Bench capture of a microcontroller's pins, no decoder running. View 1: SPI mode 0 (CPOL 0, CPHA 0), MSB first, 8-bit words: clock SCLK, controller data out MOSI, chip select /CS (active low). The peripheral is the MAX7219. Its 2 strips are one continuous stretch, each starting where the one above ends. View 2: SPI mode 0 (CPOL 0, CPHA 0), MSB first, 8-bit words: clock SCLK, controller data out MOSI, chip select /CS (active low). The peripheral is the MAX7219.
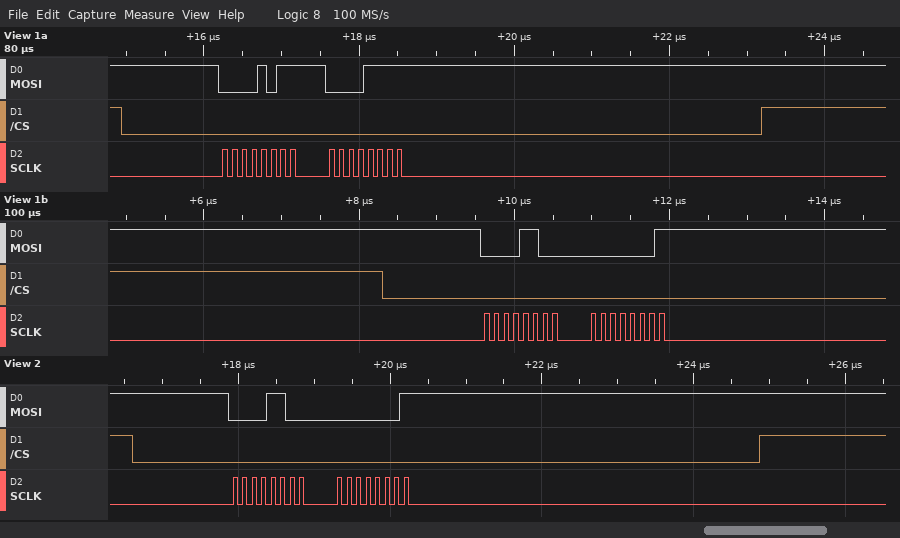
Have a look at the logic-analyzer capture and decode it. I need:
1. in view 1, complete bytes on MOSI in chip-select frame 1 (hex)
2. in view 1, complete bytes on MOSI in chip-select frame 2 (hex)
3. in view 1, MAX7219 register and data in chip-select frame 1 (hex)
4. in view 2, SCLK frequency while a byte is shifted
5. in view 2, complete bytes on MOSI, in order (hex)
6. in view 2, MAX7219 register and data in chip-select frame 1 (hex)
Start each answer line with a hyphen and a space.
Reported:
- 0x0B 0x0F
- 0x0C 0x01
- register 0xB, data 0x0F
- 8 MHz
- 0C 01
- register 0xC, data 0x01
